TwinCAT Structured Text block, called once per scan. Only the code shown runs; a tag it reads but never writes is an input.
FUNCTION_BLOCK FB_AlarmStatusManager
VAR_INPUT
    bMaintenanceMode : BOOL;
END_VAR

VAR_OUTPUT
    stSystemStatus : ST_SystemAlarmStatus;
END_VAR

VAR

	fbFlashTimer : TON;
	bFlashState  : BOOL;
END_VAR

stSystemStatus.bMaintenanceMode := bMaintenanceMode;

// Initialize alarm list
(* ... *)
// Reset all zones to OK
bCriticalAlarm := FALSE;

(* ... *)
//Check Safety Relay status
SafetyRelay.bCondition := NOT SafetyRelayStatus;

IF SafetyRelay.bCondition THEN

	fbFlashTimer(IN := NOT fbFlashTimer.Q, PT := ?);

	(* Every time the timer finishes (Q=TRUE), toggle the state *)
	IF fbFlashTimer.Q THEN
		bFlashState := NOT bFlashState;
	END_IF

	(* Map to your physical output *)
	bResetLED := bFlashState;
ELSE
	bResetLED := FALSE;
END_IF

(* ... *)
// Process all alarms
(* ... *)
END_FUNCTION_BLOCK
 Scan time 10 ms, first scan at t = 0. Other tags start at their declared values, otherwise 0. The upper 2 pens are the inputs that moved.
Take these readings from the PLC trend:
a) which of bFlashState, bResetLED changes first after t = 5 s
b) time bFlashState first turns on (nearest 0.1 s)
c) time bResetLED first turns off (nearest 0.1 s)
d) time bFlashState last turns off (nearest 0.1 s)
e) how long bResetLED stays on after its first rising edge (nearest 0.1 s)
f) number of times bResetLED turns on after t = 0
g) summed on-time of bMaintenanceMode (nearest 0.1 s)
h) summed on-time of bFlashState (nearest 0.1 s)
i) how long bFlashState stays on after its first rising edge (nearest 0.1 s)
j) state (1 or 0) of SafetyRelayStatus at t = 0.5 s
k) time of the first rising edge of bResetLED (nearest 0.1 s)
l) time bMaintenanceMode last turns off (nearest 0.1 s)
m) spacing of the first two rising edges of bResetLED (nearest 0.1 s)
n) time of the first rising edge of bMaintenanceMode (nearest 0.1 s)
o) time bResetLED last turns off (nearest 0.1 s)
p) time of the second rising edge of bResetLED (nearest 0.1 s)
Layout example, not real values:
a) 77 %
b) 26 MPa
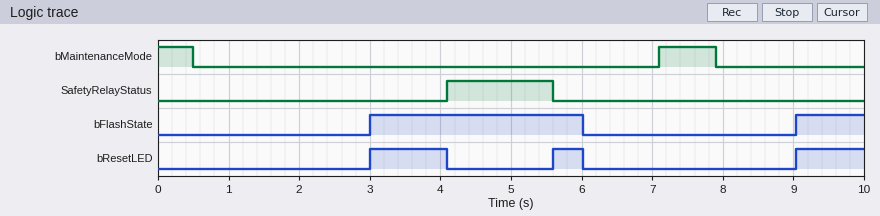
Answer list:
a) bResetLED
b) 3.0 s
c) 4.1 s
d) 6.0 s
e) 1.1 s
f) 3
g) 1.3 s
h) 4.0 s
i) 3.0 s
j) 0
k) 3.0 s
l) 7.9 s
m) 2.6 s
n) 7.1 s
o) 6.0 s
p) 5.6 s
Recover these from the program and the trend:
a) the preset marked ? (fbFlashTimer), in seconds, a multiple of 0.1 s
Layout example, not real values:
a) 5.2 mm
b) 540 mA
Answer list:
a) 3.0 s
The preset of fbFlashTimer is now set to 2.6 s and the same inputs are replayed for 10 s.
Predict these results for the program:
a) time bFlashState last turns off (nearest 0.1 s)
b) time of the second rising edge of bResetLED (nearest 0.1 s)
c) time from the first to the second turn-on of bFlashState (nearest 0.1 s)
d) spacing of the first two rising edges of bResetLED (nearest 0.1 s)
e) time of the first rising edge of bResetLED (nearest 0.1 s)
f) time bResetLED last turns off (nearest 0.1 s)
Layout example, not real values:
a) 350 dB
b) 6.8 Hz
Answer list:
a) 5.6 s
b) 8.2 s
c) 5.6 s
d) 5.6 s
e) 2.6 s
f) 4.1 s
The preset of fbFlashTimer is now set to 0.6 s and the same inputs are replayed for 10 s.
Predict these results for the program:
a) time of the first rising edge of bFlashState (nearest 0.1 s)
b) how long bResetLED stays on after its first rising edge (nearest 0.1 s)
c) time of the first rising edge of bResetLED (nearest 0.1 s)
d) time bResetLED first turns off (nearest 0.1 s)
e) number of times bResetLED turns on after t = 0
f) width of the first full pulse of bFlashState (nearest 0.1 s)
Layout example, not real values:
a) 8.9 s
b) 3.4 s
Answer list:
a) 0.6 s
b) 0.6 s
c) 0.6 s
d) 1.2 s
e) 7
f) 0.6 s
